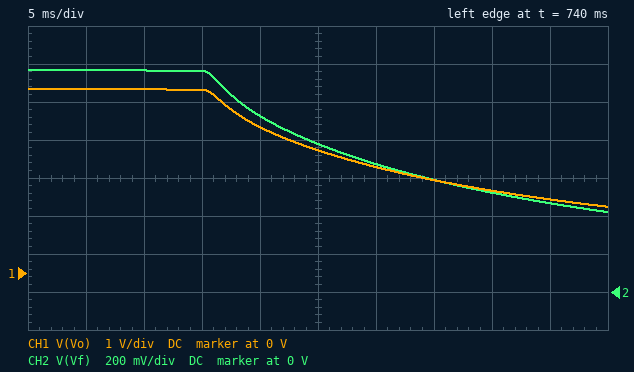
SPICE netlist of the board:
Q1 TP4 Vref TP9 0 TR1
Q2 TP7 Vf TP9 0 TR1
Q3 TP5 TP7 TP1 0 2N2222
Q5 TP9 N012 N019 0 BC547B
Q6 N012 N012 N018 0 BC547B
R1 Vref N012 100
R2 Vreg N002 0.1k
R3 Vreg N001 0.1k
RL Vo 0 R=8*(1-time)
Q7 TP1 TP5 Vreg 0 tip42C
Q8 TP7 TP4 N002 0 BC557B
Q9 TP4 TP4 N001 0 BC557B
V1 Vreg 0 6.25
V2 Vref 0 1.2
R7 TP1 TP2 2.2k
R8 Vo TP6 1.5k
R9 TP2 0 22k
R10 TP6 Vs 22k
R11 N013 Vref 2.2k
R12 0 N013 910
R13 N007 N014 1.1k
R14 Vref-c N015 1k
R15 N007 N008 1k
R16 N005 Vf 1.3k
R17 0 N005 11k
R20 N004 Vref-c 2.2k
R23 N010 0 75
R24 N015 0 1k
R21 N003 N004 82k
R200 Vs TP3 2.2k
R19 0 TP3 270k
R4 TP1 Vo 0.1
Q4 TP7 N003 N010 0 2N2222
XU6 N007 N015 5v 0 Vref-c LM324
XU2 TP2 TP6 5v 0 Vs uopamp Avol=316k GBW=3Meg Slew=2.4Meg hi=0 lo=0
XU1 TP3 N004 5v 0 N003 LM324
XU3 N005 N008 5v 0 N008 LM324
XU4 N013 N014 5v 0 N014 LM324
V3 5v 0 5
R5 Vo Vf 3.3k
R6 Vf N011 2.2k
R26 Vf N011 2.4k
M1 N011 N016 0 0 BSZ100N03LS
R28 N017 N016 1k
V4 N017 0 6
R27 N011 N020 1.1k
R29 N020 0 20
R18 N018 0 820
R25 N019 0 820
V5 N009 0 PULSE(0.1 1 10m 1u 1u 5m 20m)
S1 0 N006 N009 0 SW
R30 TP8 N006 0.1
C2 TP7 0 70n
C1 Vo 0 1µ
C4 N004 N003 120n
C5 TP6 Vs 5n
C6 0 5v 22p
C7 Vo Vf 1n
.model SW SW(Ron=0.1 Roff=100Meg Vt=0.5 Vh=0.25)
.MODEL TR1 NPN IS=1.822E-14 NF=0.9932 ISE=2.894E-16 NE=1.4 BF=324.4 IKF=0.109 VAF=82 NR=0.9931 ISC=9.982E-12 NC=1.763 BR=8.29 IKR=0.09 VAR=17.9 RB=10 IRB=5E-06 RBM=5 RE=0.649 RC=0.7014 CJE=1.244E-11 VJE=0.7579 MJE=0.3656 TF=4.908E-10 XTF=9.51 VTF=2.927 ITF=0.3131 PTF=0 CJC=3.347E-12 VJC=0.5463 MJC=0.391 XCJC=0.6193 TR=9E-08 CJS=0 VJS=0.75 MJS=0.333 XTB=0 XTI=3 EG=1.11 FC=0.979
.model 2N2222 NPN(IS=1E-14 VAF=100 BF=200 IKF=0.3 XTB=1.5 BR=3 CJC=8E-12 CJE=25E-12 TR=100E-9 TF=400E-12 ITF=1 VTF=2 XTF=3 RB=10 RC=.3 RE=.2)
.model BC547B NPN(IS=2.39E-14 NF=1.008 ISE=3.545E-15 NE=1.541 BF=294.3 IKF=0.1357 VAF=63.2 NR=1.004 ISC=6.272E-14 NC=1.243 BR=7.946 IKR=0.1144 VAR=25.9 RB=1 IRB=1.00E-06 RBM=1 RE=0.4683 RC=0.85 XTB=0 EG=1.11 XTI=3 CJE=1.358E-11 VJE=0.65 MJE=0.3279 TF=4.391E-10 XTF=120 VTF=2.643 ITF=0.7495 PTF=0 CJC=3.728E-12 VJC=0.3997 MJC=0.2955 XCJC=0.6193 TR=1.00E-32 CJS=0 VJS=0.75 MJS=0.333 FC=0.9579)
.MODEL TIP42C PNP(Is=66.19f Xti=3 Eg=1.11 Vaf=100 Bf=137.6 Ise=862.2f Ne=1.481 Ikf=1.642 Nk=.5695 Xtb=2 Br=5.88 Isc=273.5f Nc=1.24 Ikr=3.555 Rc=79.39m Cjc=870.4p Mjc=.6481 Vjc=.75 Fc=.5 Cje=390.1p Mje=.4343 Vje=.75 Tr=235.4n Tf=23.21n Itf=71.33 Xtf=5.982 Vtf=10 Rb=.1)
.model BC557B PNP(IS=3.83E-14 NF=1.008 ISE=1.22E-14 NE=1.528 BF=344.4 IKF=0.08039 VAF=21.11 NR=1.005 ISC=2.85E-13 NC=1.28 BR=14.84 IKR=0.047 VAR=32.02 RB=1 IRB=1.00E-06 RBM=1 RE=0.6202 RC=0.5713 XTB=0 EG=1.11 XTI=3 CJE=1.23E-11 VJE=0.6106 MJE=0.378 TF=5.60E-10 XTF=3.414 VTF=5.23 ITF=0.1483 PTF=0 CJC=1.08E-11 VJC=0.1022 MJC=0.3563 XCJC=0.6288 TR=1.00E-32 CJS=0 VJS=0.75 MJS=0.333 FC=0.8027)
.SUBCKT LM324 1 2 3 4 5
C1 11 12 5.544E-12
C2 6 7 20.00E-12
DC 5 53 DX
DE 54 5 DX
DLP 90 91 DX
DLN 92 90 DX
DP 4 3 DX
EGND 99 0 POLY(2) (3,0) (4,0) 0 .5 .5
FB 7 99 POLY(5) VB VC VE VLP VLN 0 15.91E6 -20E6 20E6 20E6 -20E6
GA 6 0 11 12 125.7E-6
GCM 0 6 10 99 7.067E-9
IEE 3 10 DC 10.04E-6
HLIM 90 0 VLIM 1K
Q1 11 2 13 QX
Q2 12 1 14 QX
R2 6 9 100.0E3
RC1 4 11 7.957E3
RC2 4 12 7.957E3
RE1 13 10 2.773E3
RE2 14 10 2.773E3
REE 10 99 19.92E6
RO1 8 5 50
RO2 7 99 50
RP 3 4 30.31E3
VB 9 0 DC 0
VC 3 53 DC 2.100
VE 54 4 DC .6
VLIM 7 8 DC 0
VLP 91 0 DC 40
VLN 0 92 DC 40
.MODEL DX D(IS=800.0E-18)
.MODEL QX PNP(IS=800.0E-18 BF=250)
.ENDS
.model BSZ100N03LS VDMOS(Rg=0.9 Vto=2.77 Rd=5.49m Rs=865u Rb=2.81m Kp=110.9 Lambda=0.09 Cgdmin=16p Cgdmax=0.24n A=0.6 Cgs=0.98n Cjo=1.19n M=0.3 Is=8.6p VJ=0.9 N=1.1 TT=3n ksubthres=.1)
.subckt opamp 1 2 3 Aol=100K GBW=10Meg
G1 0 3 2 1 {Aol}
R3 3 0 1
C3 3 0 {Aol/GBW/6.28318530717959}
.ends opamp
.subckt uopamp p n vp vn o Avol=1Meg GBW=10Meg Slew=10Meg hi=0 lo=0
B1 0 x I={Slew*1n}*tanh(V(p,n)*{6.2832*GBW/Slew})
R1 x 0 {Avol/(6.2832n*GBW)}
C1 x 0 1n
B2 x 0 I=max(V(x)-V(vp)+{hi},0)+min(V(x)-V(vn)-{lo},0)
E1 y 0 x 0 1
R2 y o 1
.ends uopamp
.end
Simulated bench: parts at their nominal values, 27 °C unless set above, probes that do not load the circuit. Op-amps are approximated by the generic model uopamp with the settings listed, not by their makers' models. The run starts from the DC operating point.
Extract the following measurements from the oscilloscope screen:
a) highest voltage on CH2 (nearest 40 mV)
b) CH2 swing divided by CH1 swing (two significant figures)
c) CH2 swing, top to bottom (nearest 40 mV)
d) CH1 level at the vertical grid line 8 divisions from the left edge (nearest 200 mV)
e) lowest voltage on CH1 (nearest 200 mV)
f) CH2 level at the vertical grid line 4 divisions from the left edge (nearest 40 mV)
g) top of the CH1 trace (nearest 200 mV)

1.16 V
0.24
760 mV
2.2 V
1.8 V
920 mV
4.8 V
